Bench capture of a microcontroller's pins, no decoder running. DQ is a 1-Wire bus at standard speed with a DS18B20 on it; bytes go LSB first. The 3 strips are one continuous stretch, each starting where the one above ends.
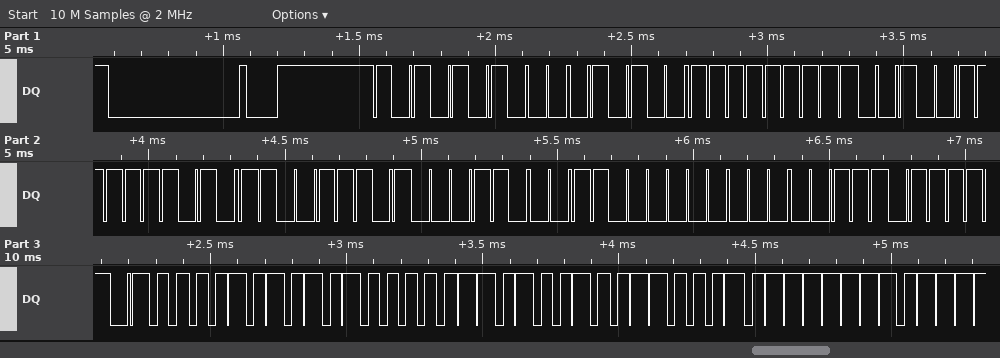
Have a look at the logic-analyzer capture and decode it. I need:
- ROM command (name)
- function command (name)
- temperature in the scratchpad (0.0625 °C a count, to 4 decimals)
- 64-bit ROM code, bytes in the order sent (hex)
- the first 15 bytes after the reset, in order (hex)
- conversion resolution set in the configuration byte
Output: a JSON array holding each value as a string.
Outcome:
["Match ROM", "Read Scratchpad", "85.0000 °C", "28 FF C9 AF B9 18 03 E0", "55 28 FF C9 AF B9 18 03 E0 BE 50 05 4B 46 7F", "12 bits"]
